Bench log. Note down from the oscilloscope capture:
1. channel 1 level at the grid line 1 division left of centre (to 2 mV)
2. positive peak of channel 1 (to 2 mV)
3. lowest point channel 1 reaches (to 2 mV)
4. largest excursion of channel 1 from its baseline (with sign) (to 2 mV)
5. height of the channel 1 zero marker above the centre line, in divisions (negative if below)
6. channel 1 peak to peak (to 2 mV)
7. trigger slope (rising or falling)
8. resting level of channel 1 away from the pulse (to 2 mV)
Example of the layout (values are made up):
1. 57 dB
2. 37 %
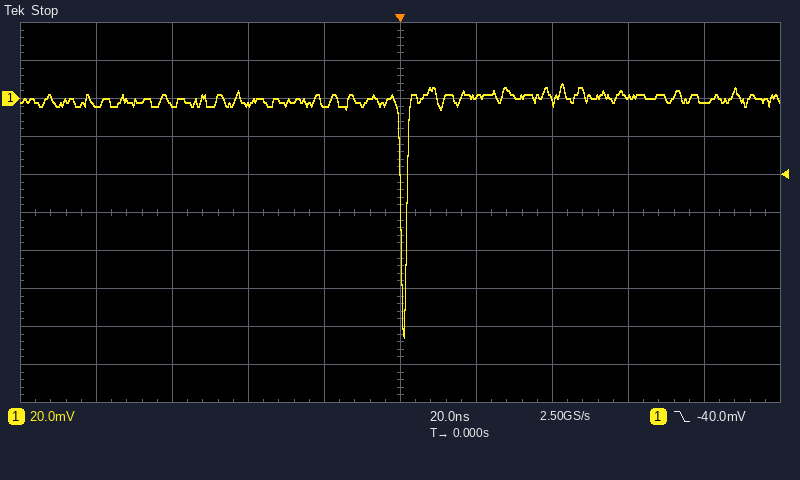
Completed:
1. -2 mV
2. 8 mV
3. -126 mV
4. -126 mV
5. +3.0 div
6. 134 mV
7. falling
8. 0 mV
